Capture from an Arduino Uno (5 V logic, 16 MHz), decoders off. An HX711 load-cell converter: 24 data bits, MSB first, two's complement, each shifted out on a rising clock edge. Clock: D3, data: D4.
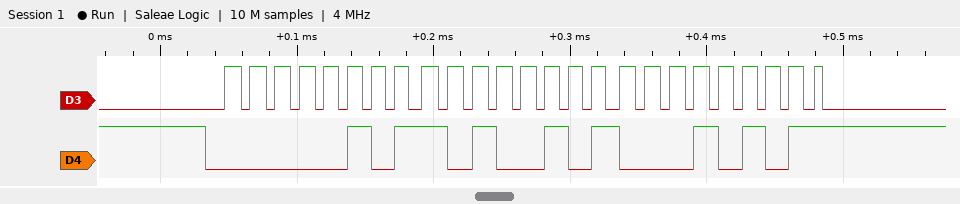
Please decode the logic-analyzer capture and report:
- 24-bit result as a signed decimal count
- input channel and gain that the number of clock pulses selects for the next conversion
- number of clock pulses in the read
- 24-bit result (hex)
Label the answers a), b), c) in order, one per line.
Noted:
a) 369941
b) channel A, gain 128
c) 25
d) 0x05A515
